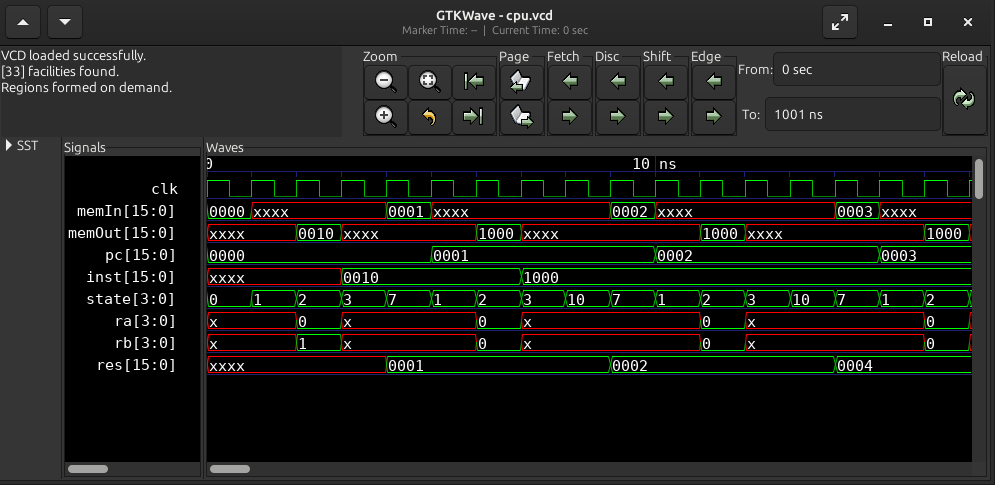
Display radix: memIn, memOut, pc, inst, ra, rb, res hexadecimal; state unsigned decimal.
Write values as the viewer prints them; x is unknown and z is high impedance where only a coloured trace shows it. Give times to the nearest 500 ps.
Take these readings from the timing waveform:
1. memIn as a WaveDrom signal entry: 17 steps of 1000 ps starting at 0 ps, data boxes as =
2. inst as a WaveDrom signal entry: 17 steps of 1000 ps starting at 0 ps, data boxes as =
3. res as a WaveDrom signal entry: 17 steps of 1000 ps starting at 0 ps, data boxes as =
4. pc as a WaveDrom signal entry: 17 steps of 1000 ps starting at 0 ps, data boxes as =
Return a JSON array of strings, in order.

["{name: 'memIn', wave: '=x..=x...=x...=x.', data: '0000 0001 0002 0003'}", "{name: 'inst', wave: 'x..=...=.........', data: '0010 1000'}", "{name: 'res', wave: 'x...=....=....=..', data: '0001 0002 0004'}", "{name: 'pc', wave: '=....=....=....=.', data: '0000 0001 0002 0003'}"]
